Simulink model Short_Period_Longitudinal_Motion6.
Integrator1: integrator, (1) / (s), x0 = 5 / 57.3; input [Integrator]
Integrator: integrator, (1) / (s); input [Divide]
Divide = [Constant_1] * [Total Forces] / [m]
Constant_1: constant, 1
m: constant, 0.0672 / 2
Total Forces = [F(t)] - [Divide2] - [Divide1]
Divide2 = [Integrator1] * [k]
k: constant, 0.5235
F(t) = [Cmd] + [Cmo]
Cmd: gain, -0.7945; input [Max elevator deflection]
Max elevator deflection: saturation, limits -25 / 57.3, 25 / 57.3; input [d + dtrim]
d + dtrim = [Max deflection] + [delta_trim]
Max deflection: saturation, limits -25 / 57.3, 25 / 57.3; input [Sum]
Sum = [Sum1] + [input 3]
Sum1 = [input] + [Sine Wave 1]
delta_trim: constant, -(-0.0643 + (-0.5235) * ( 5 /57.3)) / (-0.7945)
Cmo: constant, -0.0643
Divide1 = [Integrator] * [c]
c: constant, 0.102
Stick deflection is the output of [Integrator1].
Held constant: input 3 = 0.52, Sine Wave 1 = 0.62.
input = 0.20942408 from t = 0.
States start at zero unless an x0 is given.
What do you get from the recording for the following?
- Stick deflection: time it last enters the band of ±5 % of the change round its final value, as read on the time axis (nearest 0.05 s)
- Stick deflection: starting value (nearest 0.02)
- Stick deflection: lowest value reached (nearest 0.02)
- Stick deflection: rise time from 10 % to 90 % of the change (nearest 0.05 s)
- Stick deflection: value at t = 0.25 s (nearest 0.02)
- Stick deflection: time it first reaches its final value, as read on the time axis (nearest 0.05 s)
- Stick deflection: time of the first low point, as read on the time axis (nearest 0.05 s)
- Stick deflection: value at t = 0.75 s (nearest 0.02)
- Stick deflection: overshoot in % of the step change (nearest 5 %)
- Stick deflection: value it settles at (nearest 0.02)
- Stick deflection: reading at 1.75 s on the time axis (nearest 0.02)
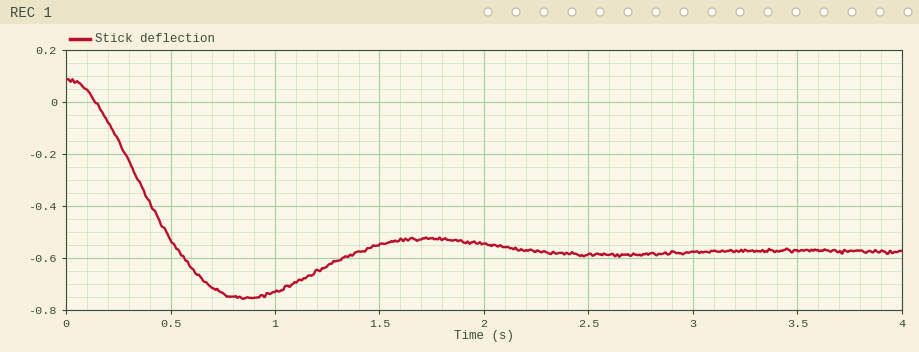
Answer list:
1.95 s
0.08
-0.76
0.35 s
-0.14
0.55 s
0.85 s
-0.74
25 %
-0.58
-0.52
